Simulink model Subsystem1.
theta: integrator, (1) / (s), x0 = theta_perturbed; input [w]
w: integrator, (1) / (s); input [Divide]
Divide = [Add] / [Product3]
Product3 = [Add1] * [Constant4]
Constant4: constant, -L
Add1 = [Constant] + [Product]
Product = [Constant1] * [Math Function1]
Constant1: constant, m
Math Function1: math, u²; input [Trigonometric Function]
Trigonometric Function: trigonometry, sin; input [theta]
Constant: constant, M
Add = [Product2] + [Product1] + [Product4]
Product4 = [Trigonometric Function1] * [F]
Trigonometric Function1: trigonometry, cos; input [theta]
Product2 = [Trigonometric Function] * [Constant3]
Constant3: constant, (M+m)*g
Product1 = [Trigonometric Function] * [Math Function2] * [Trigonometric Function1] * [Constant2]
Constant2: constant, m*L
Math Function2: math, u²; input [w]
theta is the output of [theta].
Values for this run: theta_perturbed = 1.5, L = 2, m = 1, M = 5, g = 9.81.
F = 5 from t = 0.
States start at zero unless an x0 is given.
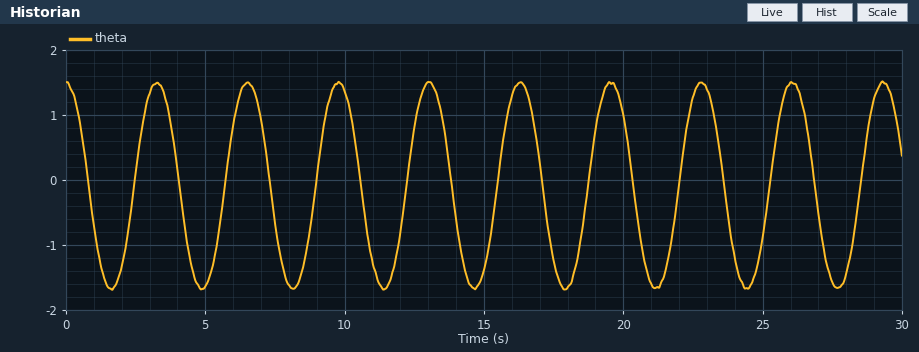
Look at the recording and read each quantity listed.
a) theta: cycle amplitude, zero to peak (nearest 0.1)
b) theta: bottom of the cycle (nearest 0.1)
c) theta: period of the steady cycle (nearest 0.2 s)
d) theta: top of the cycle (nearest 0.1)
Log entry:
1.6
-1.7
3.2 s
1.5
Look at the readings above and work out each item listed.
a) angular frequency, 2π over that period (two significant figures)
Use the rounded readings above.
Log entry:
2.0 rad/s
